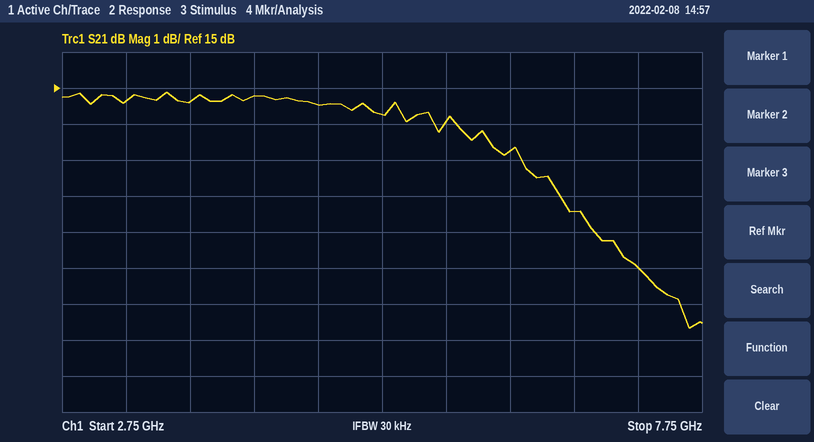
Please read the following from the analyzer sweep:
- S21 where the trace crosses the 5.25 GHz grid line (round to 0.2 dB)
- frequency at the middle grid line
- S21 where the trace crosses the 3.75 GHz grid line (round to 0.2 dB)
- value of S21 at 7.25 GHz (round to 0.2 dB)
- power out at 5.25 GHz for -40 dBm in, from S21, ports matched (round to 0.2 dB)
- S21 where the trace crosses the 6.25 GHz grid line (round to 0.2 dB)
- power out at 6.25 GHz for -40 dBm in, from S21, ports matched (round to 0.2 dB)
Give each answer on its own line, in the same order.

14.2 dB
5.25 GHz
14.6 dB
10.0 dB
-25.8 dBm
13.2 dB
-26.8 dBm
